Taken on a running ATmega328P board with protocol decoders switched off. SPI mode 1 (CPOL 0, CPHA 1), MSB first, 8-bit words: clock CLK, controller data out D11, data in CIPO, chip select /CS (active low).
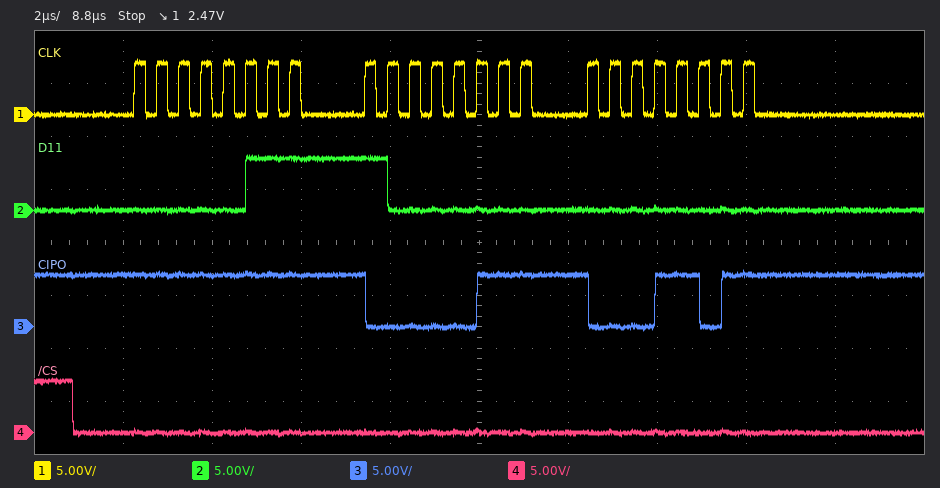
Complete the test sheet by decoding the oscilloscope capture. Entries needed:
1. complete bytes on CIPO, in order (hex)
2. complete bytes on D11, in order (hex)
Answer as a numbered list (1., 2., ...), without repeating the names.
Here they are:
1. FF 07 1B
2. 07 80 00
